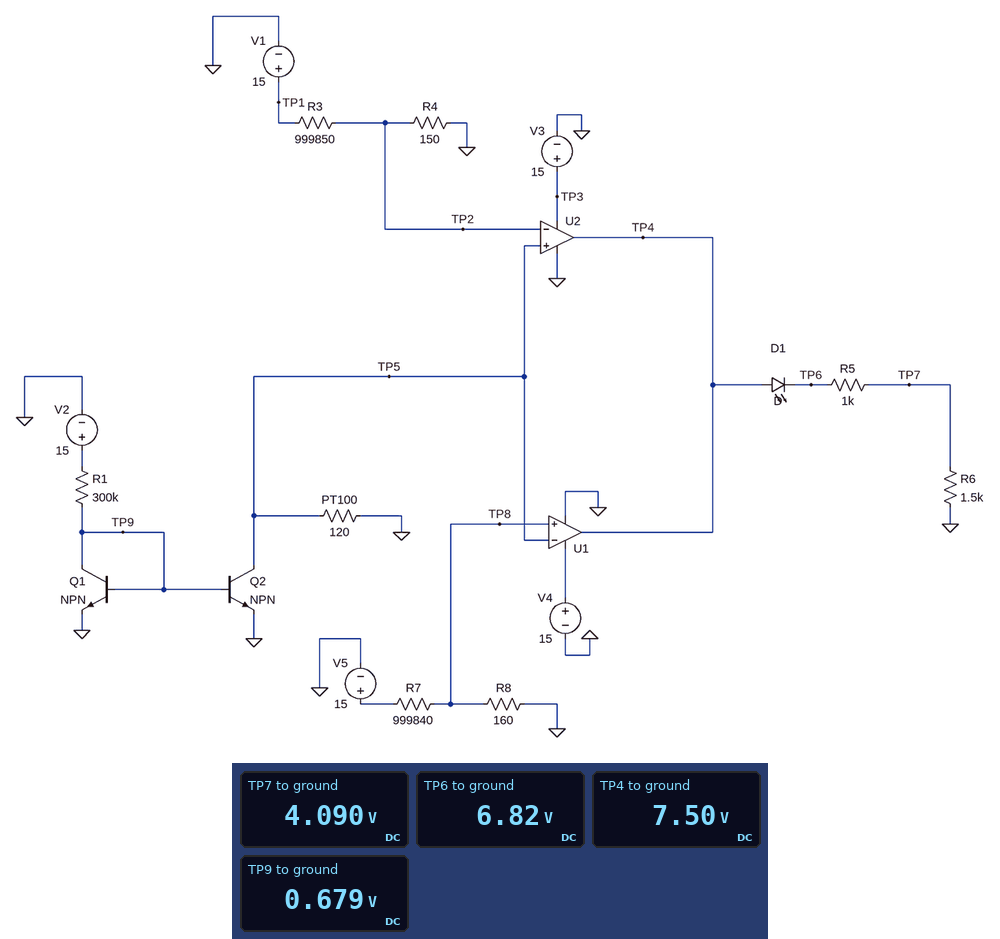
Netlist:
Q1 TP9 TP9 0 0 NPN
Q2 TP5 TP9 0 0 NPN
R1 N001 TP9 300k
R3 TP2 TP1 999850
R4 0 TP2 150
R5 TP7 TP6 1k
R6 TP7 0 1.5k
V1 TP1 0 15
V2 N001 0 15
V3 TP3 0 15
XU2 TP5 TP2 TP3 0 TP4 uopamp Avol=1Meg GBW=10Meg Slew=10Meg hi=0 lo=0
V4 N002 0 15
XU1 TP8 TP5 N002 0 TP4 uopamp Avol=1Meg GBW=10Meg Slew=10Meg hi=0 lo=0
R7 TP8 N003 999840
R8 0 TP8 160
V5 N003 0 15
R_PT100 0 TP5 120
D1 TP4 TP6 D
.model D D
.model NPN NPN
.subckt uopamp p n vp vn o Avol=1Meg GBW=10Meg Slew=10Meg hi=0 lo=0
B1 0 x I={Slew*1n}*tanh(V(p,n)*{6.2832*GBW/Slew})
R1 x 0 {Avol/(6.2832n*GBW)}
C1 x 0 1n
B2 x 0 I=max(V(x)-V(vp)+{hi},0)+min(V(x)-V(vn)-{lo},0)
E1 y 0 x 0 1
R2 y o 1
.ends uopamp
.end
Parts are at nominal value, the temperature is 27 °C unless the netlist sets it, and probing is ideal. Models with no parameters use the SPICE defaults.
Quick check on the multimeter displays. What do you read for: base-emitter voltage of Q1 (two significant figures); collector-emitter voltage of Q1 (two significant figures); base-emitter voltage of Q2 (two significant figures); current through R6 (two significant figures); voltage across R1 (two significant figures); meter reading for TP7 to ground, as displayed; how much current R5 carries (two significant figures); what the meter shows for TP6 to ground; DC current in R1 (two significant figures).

680 mV
680 mV
680 mV
2.7 mA
14 V
4.090 V
2.7 mA
6.82 V
48 µA
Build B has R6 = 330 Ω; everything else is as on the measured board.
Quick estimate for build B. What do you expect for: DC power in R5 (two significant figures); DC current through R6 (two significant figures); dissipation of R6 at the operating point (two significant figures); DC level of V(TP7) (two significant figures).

26 mW
5.1 mA
8.6 mW
1.7 V
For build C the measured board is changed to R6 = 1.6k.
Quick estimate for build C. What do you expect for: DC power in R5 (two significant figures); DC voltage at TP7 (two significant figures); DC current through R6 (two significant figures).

6.9 mW
4.2 V
2.6 mA
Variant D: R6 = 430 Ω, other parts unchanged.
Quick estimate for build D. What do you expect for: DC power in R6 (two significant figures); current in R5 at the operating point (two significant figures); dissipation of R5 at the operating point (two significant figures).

9.7 mW
4.8 mA
23 mW
